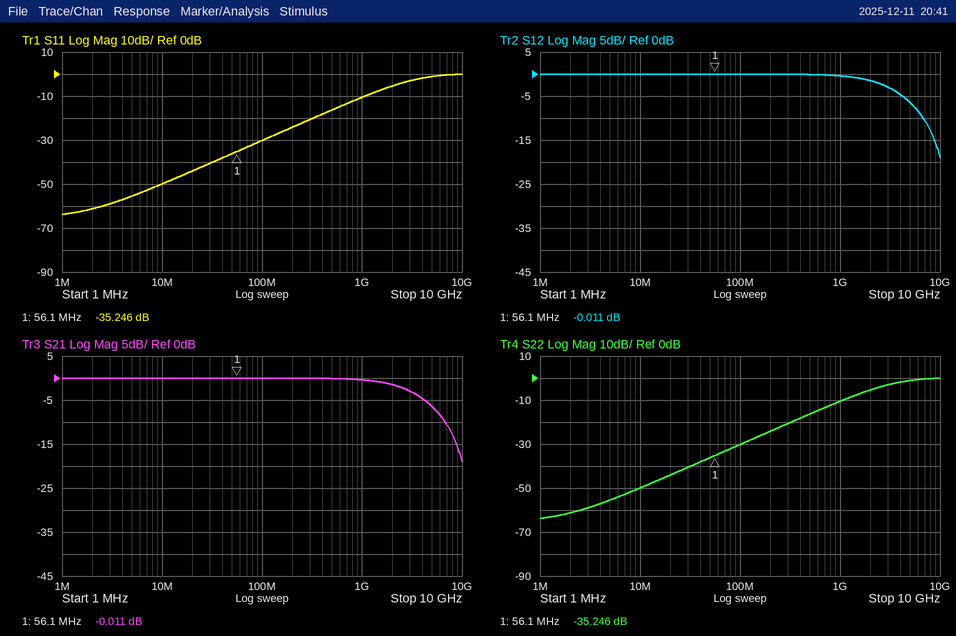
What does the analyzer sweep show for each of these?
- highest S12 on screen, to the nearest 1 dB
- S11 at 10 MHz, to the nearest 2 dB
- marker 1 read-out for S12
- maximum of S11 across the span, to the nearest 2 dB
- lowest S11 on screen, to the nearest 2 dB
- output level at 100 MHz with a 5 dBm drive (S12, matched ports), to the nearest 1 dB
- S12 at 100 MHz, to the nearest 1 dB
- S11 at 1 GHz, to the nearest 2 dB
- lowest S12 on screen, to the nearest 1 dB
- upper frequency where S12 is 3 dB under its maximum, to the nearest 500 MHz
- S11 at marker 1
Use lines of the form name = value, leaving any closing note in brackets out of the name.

highest S12 on screen, to the nearest 1 dB = 0 dB
S11 at 10 MHz, to the nearest 2 dB = -50 dB
marker 1 read-out for S12 = -0.011 dB
maximum of S11 across the span, to the nearest 2 dB = 0 dB
lowest S11 on screen, to the nearest 2 dB = -64 dB
output level at 100 MHz with a 5 dBm drive (S12, matched ports), to the nearest 1 dB = 5 dBm
S12 at 100 MHz, to the nearest 1 dB = 0 dB
S11 at 1 GHz, to the nearest 2 dB = -10 dB
lowest S12 on screen, to the nearest 1 dB = -19 dB
upper frequency where S12 is 3 dB under its maximum, to the nearest 500 MHz = 3.0 GHz
S11 at marker 1 = -35.246 dB
